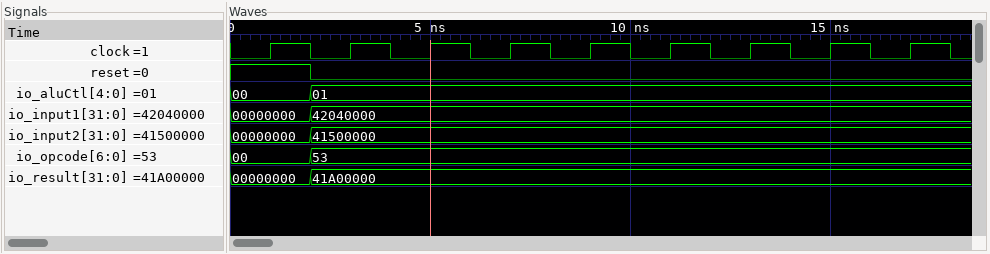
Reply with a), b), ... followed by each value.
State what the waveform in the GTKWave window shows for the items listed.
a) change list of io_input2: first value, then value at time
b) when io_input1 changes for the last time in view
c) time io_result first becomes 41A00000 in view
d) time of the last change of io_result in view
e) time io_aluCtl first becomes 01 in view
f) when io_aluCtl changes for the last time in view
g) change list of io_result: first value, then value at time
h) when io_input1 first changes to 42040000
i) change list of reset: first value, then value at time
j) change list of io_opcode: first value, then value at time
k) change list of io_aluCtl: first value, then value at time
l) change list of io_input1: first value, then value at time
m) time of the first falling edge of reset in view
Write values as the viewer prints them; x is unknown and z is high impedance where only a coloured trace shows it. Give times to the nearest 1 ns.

a) 00000000, 41500000 at 2 ns
b) 2 ns
c) 2 ns
d) 2 ns
e) 2 ns
f) 2 ns
g) 00000000, 41A00000 at 2 ns
h) 2 ns
i) 1, 0 at 2 ns
j) 00, 53 at 2 ns
k) 00, 01 at 2 ns
l) 00000000, 42040000 at 2 ns
m) 2 ns
